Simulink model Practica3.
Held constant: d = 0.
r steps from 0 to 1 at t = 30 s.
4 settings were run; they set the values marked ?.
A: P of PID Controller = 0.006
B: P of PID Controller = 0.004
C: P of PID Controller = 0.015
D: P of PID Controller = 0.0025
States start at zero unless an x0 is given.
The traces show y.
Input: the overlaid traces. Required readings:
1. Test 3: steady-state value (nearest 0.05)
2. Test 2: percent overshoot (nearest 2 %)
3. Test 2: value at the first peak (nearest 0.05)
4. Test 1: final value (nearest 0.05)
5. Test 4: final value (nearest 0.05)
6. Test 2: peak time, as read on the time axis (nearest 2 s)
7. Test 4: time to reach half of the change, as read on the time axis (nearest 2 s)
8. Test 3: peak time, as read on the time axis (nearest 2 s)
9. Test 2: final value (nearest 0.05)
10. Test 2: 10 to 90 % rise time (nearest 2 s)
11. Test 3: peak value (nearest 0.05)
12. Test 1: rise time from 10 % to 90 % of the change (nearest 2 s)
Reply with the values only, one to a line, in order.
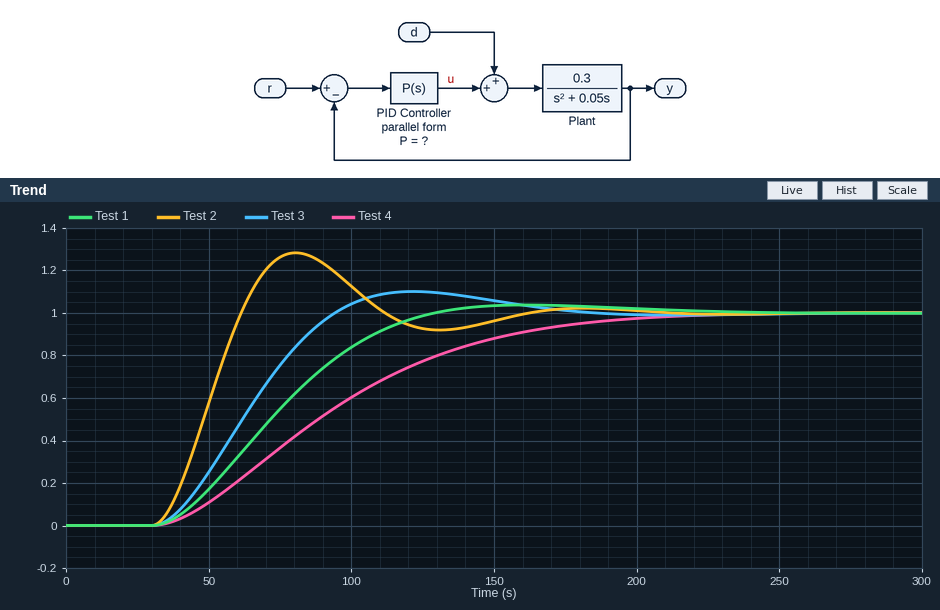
1.00
28 %
1.30
1.00
1.00
80 s
88 s
122 s
1.00
22 s
1.10
64 s
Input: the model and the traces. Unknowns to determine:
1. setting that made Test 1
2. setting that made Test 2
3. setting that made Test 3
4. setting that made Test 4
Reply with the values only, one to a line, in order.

B
C
A
D
